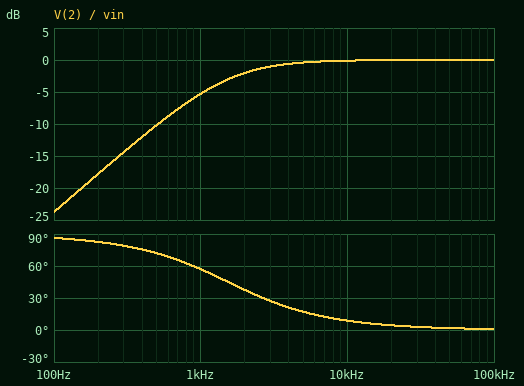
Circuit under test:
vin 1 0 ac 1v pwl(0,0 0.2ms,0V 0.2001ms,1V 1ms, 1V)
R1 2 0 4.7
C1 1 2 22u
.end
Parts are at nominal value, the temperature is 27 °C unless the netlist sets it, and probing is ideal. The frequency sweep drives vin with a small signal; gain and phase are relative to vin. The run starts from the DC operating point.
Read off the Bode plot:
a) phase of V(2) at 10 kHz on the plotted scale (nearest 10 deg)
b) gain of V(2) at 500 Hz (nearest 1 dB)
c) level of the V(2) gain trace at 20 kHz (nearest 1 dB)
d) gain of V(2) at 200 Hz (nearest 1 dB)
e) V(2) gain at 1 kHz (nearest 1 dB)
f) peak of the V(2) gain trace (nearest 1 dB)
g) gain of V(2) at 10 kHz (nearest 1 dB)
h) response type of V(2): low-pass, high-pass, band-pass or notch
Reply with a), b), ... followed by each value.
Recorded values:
a) 10 deg
b) -10 dB
c) 0 dB
d) -18 dB
e) -5 dB
f) 0 dB
g) 0 dB
h) high-pass
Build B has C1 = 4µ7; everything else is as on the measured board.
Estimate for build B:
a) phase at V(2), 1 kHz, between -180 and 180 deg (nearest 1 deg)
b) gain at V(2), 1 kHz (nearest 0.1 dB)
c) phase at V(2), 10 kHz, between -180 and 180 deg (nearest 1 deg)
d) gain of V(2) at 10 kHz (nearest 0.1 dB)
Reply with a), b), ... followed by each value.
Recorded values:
a) 82 deg
b) -17.2 dB
c) 36 deg
d) -1.8 dB
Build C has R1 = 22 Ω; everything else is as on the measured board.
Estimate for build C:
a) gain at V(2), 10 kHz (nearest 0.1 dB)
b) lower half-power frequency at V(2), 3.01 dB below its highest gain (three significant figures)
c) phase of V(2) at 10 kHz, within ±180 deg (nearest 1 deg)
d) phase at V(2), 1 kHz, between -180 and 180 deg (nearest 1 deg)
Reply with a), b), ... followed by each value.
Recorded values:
a) 0 dB
b) 329 Hz
c) 2 deg
d) 18 deg
